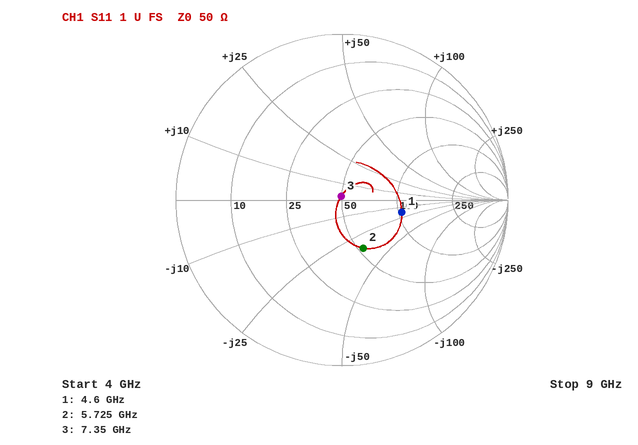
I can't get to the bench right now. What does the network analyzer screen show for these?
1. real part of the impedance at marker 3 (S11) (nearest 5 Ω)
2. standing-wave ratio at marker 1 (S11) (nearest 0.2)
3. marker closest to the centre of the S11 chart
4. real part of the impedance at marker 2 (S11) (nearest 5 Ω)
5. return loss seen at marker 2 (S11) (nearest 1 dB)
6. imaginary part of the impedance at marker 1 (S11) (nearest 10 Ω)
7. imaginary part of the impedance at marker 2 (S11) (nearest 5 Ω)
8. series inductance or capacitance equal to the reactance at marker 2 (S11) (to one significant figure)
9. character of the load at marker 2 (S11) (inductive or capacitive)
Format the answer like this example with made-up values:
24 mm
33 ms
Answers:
50 Ω
2.2
marker 3
55 Ω
10 dB
-20 Ω
-35 Ω
800 fF
capacitive
